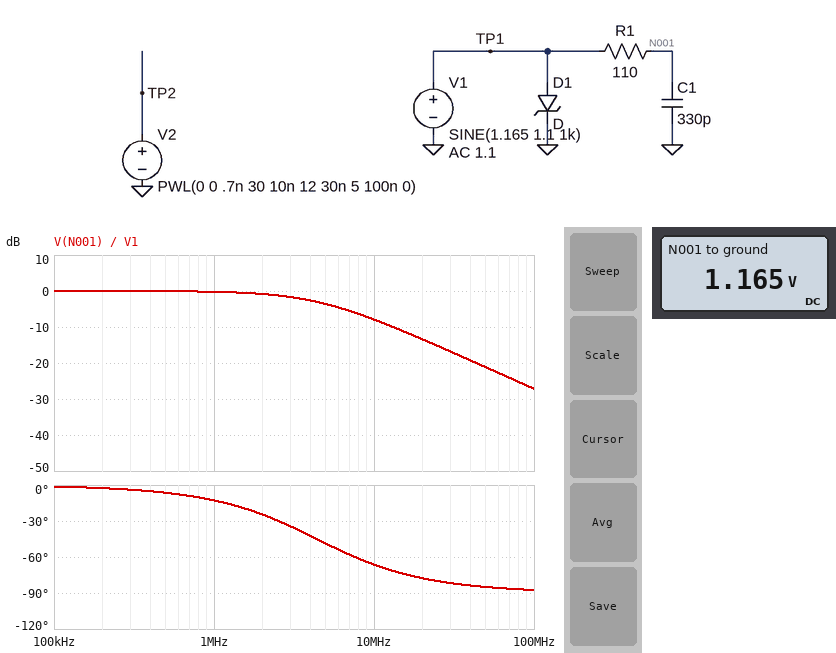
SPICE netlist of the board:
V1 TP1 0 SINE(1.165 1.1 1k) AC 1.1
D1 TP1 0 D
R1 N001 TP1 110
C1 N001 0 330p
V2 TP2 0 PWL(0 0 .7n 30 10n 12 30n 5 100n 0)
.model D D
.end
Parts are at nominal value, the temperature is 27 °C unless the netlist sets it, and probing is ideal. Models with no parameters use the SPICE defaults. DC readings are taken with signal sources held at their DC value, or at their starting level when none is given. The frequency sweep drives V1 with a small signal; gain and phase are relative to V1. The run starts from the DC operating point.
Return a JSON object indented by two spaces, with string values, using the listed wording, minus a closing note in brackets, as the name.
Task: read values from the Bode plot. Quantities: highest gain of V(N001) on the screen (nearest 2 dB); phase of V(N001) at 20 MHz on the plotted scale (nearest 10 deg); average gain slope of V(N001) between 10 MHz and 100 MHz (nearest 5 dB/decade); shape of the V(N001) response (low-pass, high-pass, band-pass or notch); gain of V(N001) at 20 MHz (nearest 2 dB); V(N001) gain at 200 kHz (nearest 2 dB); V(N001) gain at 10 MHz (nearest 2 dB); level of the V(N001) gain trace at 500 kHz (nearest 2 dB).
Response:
{
  "highest gain of V(N001) on the screen": "0 dB",
  "phase of V(N001) at 20 MHz on the plotted scale": "-80 deg",
  "average gain slope of V(N001) between 10 MHz and 100 MHz": "-20 dB/decade",
  "shape of the V(N001) response": "low-pass",
  "gain of V(N001) at 20 MHz": "-14 dB",
  "V(N001) gain at 200 kHz": "0 dB",
  "V(N001) gain at 10 MHz": "-8 dB",
  "level of the V(N001) gain trace at 500 kHz": "0 dB"
}
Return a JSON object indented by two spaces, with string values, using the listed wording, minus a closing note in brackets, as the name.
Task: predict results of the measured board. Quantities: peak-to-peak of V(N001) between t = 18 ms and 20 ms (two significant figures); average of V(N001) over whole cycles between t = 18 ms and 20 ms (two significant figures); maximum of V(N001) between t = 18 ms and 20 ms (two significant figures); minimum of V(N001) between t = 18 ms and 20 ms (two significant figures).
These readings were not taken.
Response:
{
  "peak-to-peak of V(N001) between t = 18 ms and 20 ms": "2.2 V",
  "average of V(N001) over whole cycles between t = 18 ms and 20 ms": "1.2 V",
  "maximum of V(N001) between t = 18 ms and 20 ms": "2.3 V",
  "minimum of V(N001) between t = 18 ms and 20 ms": "65 mV"
}
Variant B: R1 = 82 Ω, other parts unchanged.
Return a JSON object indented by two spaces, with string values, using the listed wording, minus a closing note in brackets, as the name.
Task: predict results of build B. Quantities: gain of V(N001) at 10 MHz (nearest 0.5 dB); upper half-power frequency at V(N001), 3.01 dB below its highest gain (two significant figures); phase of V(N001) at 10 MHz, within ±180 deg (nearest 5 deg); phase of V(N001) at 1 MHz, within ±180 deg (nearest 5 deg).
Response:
{
  "gain of V(N001) at 10 MHz": "-6.0 dB",
  "upper half-power frequency at V(N001), 3.01 dB below its highest gain": "5.9 MHz",
  "phase of V(N001) at 10 MHz, within ±180 deg": "-60 deg",
  "phase of V(N001) at 1 MHz, within ±180 deg": "-10 deg"
}
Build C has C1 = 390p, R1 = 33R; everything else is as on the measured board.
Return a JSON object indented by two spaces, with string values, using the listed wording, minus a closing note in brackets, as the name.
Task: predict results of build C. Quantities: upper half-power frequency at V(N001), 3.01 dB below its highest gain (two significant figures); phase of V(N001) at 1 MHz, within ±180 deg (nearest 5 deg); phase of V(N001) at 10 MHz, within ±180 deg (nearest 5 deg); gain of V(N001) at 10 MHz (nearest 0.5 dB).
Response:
{
  "upper half-power frequency at V(N001), 3.01 dB below its highest gain": "12 MHz",
  "phase of V(N001) at 1 MHz, within ±180 deg": "-5 deg",
  "phase of V(N001) at 10 MHz, within ±180 deg": "-40 deg",
  "gain of V(N001) at 10 MHz": "-2.0 dB"
}
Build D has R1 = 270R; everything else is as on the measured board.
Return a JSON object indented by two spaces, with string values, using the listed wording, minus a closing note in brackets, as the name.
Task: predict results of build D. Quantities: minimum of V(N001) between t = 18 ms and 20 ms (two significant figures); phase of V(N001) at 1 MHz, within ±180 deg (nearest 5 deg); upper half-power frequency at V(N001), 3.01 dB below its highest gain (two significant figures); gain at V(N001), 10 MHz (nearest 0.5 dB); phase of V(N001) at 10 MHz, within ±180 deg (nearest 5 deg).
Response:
{
  "minimum of V(N001) between t = 18 ms and 20 ms": "65 mV",
  "phase of V(N001) at 1 MHz, within ±180 deg": "-30 deg",
  "upper half-power frequency at V(N001), 3.01 dB below its highest gain": "1.8 MHz",
  "gain at V(N001), 10 MHz": "-15.0 dB",
  "phase of V(N001) at 10 MHz, within ±180 deg": "-80 deg"
}
